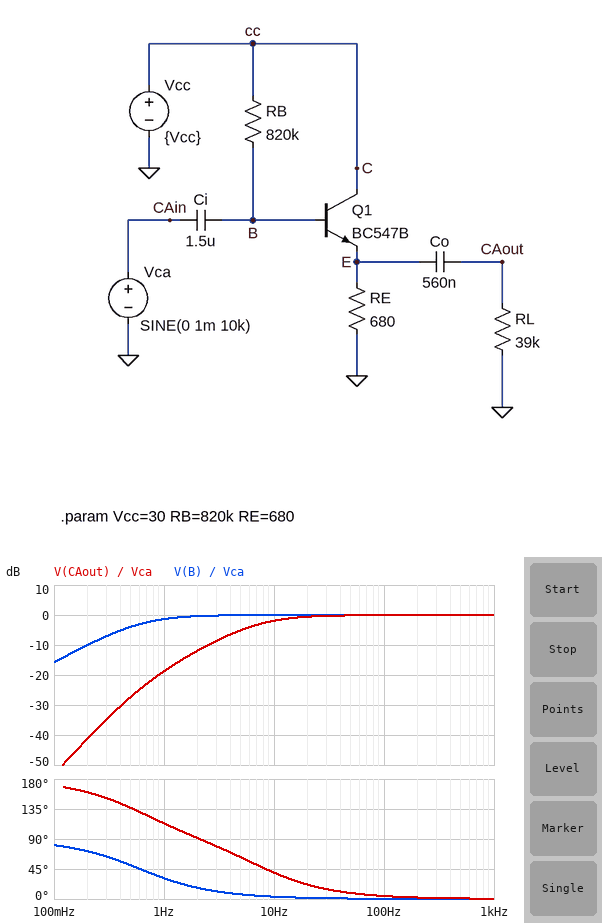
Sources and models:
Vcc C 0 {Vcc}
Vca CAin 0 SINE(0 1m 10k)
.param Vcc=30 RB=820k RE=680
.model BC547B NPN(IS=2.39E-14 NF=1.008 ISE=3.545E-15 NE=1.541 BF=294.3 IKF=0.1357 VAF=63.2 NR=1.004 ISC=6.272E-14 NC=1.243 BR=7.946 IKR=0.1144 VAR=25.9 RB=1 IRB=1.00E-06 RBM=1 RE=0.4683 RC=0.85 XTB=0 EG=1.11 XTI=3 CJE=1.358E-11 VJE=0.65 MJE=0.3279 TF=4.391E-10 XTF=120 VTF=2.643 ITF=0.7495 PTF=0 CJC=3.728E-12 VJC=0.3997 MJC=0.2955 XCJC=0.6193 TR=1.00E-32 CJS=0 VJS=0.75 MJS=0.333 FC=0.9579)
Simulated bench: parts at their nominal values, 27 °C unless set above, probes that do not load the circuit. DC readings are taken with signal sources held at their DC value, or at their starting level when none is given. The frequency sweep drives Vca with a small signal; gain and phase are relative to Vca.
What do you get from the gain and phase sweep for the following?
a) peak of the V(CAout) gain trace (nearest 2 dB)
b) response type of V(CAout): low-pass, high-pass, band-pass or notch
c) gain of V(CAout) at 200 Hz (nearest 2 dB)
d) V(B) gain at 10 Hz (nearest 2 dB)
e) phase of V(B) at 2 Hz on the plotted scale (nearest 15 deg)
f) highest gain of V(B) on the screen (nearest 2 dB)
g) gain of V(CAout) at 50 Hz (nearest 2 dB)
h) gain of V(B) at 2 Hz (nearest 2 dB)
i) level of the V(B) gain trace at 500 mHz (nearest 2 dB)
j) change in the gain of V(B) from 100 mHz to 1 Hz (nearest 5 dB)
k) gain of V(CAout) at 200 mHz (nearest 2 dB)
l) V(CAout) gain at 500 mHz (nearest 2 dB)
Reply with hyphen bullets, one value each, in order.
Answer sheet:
- 0 dB
- high-pass
- 0 dB
- 0 dB
- 15 deg
- 0 dB
- 0 dB
- 0 dB
- -4 dB
- 15 dB
- -42 dB
- -28 dB
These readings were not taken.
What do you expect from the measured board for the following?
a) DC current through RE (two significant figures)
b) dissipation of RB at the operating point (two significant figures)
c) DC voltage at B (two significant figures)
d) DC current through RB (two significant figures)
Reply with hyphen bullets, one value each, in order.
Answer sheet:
- 10 mA
- 610 µW
- 7.6 V
- 27 µA
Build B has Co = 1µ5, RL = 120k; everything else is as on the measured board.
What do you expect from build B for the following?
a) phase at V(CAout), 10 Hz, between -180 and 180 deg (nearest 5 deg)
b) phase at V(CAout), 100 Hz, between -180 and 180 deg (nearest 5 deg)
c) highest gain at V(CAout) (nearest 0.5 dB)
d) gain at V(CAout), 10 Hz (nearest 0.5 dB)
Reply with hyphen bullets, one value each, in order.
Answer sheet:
- 10 deg
- 0 deg
- 0 dB
- 0 dB
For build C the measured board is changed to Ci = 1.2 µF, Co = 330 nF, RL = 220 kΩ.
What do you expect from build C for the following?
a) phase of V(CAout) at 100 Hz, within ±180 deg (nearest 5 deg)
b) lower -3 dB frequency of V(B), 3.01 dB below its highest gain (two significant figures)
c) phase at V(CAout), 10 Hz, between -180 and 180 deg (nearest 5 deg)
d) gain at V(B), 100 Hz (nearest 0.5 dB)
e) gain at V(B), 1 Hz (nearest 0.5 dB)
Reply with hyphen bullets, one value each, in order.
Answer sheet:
- 0 deg
- 760 mHz
- 15 deg
- 0 dB
- -2.0 dB
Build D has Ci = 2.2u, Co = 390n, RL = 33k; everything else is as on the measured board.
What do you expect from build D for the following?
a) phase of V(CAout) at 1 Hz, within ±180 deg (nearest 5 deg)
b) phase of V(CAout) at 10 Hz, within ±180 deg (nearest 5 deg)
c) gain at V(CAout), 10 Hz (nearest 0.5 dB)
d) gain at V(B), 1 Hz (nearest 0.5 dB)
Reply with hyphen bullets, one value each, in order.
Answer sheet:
- 110 deg
- 55 deg
- -4.0 dB
- -0.5 dB
